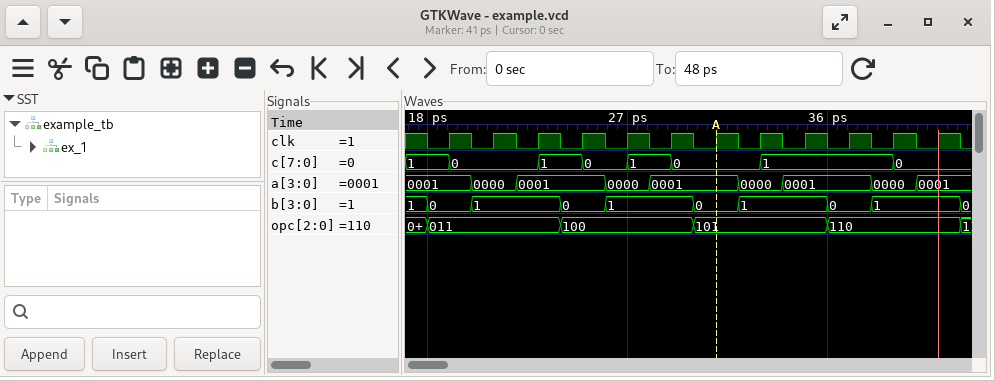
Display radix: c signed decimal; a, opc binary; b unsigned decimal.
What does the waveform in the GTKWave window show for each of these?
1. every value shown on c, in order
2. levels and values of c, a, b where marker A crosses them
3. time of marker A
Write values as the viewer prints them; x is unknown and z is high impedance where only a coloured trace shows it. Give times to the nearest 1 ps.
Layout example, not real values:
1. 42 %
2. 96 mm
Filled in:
1. 1, 0, 1, 0, 1, 0, 1, 0
2. c=0, a=0001, b=0
3. 31 ps
